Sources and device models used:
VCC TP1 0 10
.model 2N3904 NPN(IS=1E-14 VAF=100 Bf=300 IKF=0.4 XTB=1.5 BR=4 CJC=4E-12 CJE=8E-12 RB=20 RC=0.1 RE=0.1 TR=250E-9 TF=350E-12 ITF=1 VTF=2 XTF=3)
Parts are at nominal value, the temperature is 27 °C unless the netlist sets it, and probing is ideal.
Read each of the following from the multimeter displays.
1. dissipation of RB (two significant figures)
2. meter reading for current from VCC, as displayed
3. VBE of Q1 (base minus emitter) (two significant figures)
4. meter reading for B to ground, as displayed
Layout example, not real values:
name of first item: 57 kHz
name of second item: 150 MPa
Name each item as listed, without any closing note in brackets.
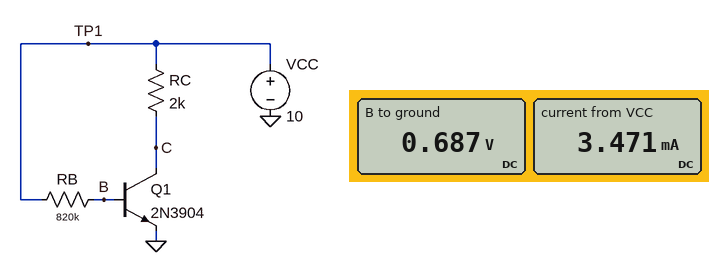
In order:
dissipation of RB: 110 µW
meter reading for current from VCC, as displayed: 3.471 mA
VBE of Q1 (base minus emitter): 690 mV
meter reading for B to ground, as displayed: 0.687 V
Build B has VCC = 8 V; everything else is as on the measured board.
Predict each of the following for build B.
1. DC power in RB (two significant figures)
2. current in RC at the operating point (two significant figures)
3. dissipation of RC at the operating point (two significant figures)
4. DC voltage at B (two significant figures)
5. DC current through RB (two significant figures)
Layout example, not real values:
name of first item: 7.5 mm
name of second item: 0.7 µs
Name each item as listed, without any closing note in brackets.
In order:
DC power in RB: 65 µW
current in RC at the operating point: 2.7 mA
dissipation of RC at the operating point: 15 mW
DC voltage at B: 680 mV
DC current through RB: 8.9 µA
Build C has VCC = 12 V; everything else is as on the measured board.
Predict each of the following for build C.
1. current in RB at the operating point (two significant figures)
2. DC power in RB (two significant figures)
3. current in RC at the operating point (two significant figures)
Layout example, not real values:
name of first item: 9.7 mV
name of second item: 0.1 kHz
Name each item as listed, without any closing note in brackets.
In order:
current in RB at the operating point: 14 µA
DC power in RB: 160 µW
current in RC at the operating point: 4.2 mA
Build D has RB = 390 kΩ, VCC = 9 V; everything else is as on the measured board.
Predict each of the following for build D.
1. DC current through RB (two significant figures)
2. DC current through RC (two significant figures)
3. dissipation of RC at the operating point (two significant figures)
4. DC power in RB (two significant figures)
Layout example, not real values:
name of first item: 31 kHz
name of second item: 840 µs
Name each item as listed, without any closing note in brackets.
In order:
DC current through RB: 21 µA
DC current through RC: 4.4 mA
dissipation of RC at the operating point: 39 mW
DC power in RB: 180 µW
